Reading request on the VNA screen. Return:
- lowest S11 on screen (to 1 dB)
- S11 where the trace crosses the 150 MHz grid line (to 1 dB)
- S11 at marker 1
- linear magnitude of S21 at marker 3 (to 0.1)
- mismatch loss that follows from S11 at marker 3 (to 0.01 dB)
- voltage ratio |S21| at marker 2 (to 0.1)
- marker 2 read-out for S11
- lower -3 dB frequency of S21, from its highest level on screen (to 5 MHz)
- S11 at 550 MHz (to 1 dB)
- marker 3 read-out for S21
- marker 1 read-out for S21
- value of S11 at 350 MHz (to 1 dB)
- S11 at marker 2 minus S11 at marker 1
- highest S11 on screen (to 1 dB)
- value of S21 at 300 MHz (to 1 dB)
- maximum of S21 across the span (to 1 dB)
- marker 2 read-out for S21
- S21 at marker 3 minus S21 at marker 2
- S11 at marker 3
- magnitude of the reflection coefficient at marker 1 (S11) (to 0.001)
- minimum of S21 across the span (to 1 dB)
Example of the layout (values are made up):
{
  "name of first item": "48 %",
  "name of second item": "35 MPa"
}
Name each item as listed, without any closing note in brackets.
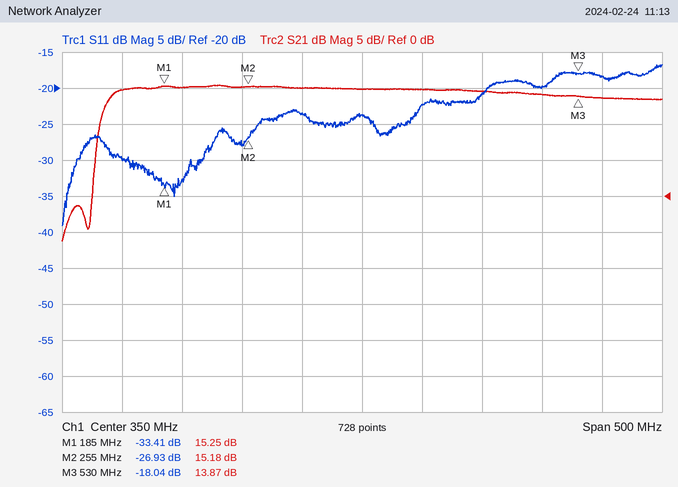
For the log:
{
  "lowest S11 on screen": "-39 dB",
  "S11 where the trace crosses the 150 MHz grid line": "-30 dB",
  "S11 at marker 1": "-33.41 dB",
  "linear magnitude of S21 at marker 3": "4.9",
  "mismatch loss that follows from S11 at marker 3": "0.07 dB",
  "voltage ratio |S21| at marker 2": "5.7",
  "marker 2 read-out for S11": "-26.93 dB",
  "lower -3 dB frequency of S21, from its highest level on screen": "135 MHz",
  "S11 at 550 MHz": "-18 dB",
  "marker 3 read-out for S21": "13.87 dB",
  "marker 1 read-out for S21": "15.25 dB",
  "value of S11 at 350 MHz": "-24 dB",
  "S11 at marker 2 minus S11 at marker 1": "6.48 dB",
  "highest S11 on screen": "-17 dB",
  "value of S21 at 300 MHz": "15 dB",
  "maximum of S21 across the span": "15 dB",
  "marker 2 read-out for S21": "15.18 dB",
  "S21 at marker 3 minus S21 at marker 2": "-1.31 dB",
  "S11 at marker 3": "-18.04 dB",
  "magnitude of the reflection coefficient at marker 1 (S11)": "0.021",
  "minimum of S21 across the span": "-6 dB"
}
